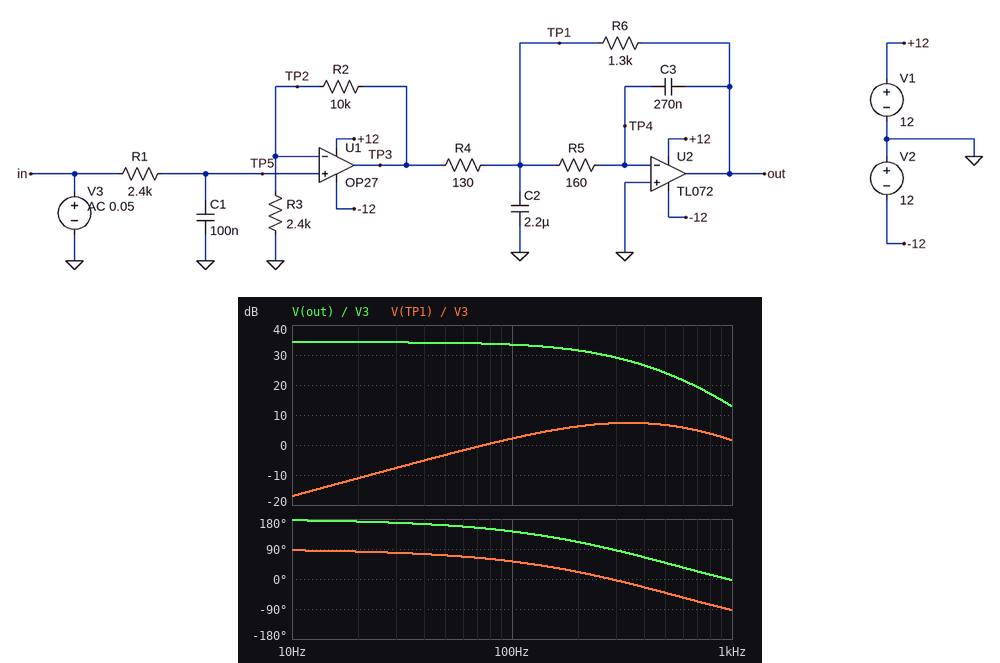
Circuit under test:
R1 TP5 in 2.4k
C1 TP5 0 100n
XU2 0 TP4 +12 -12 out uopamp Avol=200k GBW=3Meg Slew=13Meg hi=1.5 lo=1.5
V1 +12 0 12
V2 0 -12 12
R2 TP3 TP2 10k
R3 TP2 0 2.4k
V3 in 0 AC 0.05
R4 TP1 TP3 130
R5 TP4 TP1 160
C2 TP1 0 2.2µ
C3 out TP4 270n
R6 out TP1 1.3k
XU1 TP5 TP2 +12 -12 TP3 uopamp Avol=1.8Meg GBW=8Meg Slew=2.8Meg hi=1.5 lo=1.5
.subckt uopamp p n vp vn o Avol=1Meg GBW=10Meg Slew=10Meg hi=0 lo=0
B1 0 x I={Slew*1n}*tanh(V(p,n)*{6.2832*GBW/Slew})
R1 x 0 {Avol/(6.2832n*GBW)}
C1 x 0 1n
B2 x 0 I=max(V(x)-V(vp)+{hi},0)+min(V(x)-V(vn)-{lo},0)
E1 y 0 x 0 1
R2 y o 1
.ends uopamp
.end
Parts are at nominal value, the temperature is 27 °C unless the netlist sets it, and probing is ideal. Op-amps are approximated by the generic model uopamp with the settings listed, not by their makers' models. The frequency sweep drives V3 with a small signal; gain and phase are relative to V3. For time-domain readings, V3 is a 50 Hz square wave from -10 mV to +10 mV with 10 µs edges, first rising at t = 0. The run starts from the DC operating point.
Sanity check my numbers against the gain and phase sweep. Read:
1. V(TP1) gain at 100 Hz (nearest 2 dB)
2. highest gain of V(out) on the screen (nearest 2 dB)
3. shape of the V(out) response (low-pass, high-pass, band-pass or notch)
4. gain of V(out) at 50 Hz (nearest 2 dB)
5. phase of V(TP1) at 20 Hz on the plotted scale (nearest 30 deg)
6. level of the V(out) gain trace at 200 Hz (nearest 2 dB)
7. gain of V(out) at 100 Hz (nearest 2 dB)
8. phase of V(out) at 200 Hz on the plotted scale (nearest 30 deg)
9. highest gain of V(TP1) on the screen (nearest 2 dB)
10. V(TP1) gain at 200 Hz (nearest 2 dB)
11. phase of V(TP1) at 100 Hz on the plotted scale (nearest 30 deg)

2 dB
34 dB
low-pass
34 dB
90 deg
32 dB
34 dB
120 deg
8 dB
6 dB
60 deg
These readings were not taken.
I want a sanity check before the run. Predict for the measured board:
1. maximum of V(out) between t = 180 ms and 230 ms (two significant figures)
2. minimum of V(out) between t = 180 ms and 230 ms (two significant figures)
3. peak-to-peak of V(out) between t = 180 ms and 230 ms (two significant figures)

520 mV
-520 mV
1.0 V
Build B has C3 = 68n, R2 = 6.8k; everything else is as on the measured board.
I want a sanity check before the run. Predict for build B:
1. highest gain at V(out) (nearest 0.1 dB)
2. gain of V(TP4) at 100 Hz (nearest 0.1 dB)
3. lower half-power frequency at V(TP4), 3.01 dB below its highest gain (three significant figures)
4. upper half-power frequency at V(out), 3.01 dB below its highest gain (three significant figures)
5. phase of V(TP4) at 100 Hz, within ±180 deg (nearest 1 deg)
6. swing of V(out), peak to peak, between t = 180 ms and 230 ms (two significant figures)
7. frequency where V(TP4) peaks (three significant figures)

31.7 dB
-57.8 dB
378 Hz
678 Hz
65 deg
790 mV
730 Hz
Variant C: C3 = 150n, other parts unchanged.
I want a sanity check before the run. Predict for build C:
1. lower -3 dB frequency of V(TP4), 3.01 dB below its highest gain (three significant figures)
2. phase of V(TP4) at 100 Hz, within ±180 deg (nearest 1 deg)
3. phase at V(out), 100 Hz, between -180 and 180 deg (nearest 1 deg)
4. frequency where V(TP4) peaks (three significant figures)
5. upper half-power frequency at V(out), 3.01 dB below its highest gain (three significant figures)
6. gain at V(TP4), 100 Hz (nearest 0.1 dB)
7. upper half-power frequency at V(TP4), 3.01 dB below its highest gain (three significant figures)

216 Hz
56 deg
155 deg
465 Hz
368 Hz
-55.4 dB
878 Hz
